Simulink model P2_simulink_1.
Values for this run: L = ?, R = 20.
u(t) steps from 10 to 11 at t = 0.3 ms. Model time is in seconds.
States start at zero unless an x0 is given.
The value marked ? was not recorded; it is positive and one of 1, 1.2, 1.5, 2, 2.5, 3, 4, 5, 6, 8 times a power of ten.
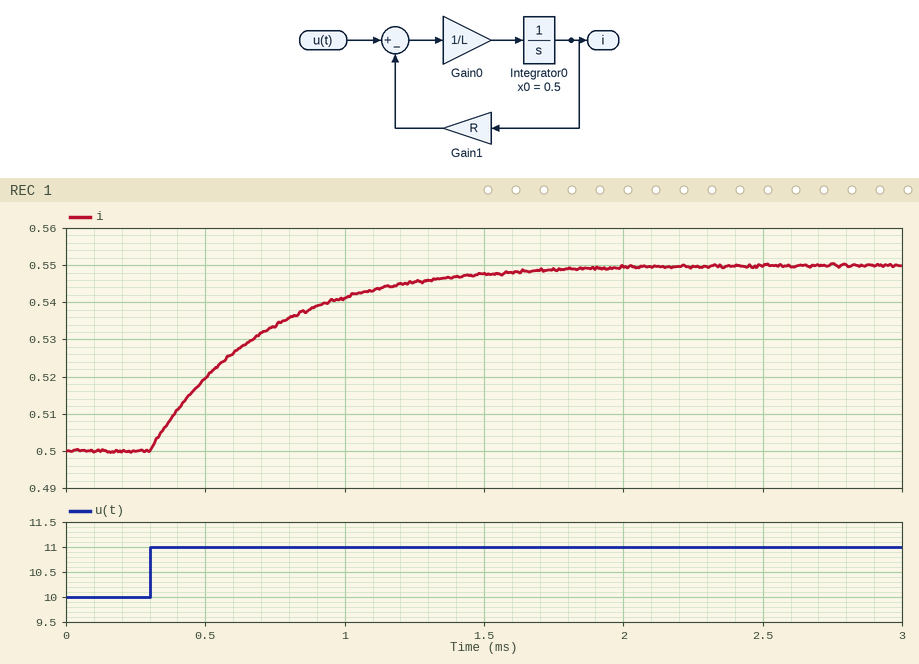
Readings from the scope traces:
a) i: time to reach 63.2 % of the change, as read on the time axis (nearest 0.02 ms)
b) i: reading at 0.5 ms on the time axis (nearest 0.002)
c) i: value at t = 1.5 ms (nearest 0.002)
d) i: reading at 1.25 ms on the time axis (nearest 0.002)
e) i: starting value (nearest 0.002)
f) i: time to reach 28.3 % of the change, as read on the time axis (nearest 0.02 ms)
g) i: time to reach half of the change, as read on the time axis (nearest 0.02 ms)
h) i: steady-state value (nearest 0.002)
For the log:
0.70 ms
0.520
0.548
0.546
0.500
0.44 ms
0.58 ms
0.550
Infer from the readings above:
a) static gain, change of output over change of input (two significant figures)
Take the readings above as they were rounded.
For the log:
0.050
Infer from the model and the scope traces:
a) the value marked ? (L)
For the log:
0.008
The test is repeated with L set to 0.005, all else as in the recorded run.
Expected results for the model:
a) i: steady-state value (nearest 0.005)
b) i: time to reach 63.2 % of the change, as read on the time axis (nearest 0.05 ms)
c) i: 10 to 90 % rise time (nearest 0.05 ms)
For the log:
0.550
0.55 ms
0.55 ms
